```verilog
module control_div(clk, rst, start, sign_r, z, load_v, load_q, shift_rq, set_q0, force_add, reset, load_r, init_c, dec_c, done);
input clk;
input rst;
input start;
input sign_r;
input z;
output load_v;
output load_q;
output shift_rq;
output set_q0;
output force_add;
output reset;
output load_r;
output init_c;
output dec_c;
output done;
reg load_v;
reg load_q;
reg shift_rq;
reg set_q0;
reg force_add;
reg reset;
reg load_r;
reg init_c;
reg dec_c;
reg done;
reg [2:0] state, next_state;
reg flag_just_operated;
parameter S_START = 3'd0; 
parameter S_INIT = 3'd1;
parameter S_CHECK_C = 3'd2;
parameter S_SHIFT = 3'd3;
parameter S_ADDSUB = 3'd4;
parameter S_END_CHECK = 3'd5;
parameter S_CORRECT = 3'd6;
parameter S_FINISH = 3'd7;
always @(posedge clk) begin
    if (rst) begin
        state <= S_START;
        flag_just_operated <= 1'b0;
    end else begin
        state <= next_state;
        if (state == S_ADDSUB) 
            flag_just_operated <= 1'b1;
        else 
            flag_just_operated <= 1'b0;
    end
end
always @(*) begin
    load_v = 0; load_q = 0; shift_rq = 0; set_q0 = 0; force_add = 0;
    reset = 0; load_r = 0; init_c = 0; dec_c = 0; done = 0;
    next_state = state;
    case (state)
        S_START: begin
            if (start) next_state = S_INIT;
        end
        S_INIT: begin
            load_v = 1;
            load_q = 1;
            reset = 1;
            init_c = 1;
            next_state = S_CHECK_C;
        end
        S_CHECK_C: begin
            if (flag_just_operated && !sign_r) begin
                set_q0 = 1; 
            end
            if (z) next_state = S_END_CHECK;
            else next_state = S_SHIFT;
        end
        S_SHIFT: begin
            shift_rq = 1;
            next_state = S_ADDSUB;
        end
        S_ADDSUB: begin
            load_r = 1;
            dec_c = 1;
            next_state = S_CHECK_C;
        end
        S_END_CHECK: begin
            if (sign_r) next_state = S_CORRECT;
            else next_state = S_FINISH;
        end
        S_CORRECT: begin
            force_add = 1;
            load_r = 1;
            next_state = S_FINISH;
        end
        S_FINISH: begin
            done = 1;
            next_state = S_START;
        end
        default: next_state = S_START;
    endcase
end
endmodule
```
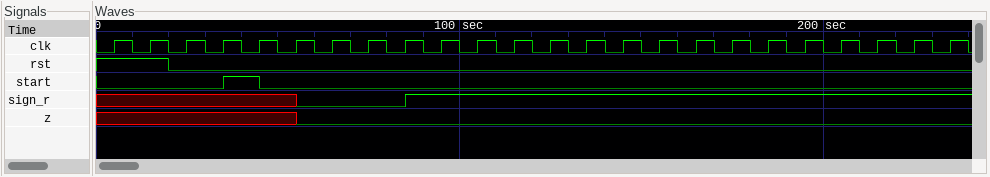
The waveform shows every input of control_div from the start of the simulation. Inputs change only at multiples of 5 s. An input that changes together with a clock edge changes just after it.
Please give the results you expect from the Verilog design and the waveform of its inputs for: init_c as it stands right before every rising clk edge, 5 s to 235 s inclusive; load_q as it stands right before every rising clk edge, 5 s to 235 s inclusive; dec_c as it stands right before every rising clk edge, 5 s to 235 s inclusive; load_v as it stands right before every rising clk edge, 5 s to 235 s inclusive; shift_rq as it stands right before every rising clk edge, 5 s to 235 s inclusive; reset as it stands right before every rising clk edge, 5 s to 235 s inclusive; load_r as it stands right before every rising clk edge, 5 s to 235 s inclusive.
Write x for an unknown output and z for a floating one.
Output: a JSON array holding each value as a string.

["0 0 0 0 0 1 0 0 0 0 0 0 0 0 0 0 0 0 0 0 0 0 0 0", "0 0 0 0 0 1 0 0 0 0 0 0 0 0 0 0 0 0 0 0 0 0 0 0", "0 0 0 0 0 0 0 0 1 0 0 1 0 0 1 0 0 1 0 0 1 0 0 1", "0 0 0 0 0 1 0 0 0 0 0 0 0 0 0 0 0 0 0 0 0 0 0 0", "0 0 0 0 0 0 0 1 0 0 1 0 0 1 0 0 1 0 0 1 0 0 1 0", "0 0 0 0 0 1 0 0 0 0 0 0 0 0 0 0 0 0 0 0 0 0 0 0", "0 0 0 0 0 0 0 0 1 0 0 1 0 0 1 0 0 1 0 0 1 0 0 1"]
